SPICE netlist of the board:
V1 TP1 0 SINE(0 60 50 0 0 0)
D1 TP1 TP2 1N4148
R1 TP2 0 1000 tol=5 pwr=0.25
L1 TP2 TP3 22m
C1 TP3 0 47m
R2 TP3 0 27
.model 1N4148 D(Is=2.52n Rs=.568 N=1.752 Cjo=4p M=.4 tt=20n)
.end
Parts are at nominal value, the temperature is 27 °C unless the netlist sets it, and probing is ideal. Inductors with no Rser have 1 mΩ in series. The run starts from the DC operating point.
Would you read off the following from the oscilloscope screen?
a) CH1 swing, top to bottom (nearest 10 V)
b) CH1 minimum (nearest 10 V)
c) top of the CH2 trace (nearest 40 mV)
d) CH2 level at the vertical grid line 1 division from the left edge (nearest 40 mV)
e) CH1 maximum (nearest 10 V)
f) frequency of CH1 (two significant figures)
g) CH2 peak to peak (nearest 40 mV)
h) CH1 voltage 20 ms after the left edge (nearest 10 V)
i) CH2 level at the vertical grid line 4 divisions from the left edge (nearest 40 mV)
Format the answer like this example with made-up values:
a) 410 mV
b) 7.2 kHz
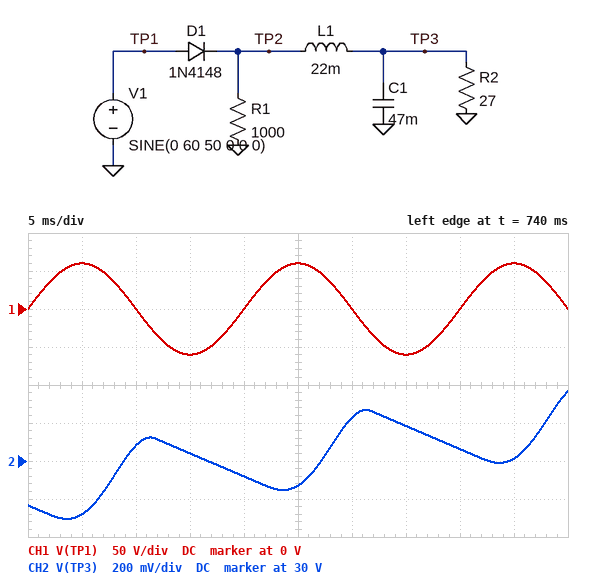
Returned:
a) 120 V
b) -60 V
c) 30.36 V
d) 29.72 V
e) 60 V
f) 50 Hz
g) 680 mV
h) 0 V
i) 29.92 V
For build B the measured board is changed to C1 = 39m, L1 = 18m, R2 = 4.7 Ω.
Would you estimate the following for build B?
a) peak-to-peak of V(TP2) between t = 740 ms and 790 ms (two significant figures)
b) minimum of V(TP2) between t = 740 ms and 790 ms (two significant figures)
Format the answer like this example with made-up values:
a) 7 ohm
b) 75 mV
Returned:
a) 110 V
b) -53 V
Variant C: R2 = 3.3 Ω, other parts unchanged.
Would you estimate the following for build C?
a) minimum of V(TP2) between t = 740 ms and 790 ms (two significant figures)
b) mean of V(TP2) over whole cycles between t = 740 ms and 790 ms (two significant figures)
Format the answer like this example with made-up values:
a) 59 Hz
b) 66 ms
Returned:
a) -59 V
b) 13 V
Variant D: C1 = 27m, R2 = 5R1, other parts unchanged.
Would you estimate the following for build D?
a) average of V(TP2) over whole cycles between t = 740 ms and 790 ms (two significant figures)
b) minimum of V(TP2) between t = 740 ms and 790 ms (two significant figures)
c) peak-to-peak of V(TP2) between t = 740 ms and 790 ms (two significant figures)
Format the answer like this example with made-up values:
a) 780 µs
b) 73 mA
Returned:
a) 17 V
b) -55 V
c) 110 V
